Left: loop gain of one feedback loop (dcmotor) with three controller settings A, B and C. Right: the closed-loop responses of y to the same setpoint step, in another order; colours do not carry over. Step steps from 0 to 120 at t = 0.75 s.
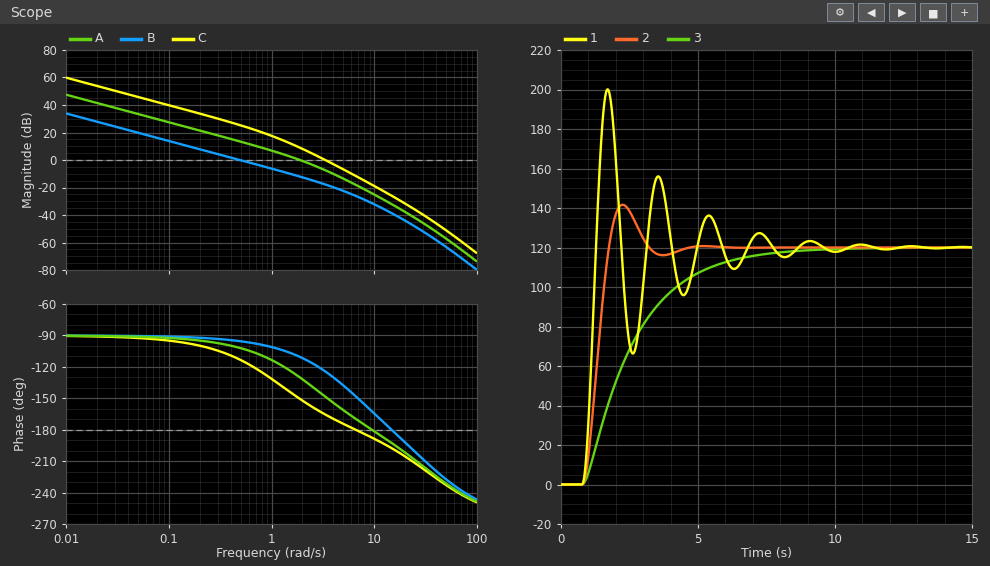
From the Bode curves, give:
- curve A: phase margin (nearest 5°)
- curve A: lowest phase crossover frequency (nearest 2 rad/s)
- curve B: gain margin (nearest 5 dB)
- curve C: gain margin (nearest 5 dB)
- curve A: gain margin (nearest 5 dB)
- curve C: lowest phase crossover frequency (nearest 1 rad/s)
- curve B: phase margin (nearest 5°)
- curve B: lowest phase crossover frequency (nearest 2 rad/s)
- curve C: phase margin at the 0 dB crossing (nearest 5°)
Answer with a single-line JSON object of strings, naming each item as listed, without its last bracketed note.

{"curve A: phase margin": "50°", "curve A: lowest phase crossover frequency": "10 rad/s", "curve B: gain margin": "40 dB", "curve C: gain margin": "10 dB", "curve A: gain margin": "25 dB", "curve C: lowest phase crossover frequency": "7 rad/s", "curve B: phase margin": "85°", "curve B: lowest phase crossover frequency": "14 rad/s", "curve C: phase margin at the 0 dB crossing": "15°"}
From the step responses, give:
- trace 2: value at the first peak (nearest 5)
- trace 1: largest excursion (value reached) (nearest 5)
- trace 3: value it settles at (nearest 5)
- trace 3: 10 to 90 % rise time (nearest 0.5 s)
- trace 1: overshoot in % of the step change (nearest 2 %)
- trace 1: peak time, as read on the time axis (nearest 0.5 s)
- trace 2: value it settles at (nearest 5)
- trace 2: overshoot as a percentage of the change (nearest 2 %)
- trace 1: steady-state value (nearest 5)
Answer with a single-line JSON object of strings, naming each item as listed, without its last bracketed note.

{"trace 2: value at the first peak": "140", "trace 1: largest excursion (value reached)": "200", "trace 3: value it settles at": "120", "trace 3: 10 to 90 % rise time": "4.0 s", "trace 1: overshoot in % of the step change": "66 %", "trace 1: peak time, as read on the time axis": "1.5 s", "trace 2: value it settles at": "120", "trace 2: overshoot as a percentage of the change": "18 %", "trace 1: steady-state value": "120"}
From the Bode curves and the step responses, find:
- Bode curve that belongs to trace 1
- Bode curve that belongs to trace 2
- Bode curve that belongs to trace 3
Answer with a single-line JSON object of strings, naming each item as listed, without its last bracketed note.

{"Bode curve that belongs to trace 1": "C", "Bode curve that belongs to trace 2": "A", "Bode curve that belongs to trace 3": "B"}
